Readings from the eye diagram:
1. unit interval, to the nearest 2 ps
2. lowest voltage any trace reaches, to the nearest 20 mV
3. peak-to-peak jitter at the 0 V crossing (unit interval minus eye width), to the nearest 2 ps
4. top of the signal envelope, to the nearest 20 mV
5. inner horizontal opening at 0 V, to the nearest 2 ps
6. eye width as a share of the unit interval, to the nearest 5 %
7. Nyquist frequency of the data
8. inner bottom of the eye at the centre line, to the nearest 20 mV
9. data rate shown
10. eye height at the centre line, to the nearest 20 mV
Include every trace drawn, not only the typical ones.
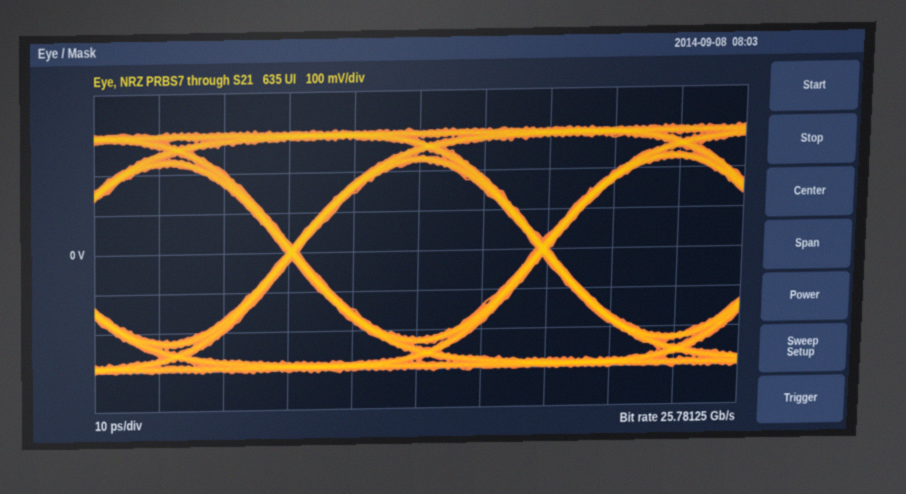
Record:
38 ps
-300 mV
2 ps
300 mV
36 ps
95 %
12.89062 GHz
-220 mV
25.78125 Gb/s
440 mV
